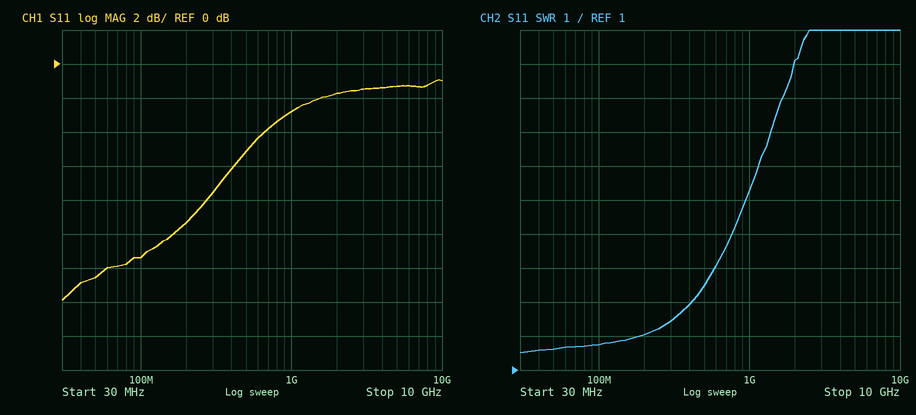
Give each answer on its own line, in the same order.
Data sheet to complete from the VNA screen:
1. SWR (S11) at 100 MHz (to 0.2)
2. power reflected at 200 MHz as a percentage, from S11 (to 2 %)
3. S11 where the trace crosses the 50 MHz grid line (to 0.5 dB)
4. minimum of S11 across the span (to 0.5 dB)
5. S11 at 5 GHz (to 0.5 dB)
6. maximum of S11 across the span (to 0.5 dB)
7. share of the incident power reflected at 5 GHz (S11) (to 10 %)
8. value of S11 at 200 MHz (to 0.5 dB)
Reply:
1.8
12 %
-12.5 dB
-14.0 dB
-1.5 dB
-1.0 dB
70 %
-9.5 dB
